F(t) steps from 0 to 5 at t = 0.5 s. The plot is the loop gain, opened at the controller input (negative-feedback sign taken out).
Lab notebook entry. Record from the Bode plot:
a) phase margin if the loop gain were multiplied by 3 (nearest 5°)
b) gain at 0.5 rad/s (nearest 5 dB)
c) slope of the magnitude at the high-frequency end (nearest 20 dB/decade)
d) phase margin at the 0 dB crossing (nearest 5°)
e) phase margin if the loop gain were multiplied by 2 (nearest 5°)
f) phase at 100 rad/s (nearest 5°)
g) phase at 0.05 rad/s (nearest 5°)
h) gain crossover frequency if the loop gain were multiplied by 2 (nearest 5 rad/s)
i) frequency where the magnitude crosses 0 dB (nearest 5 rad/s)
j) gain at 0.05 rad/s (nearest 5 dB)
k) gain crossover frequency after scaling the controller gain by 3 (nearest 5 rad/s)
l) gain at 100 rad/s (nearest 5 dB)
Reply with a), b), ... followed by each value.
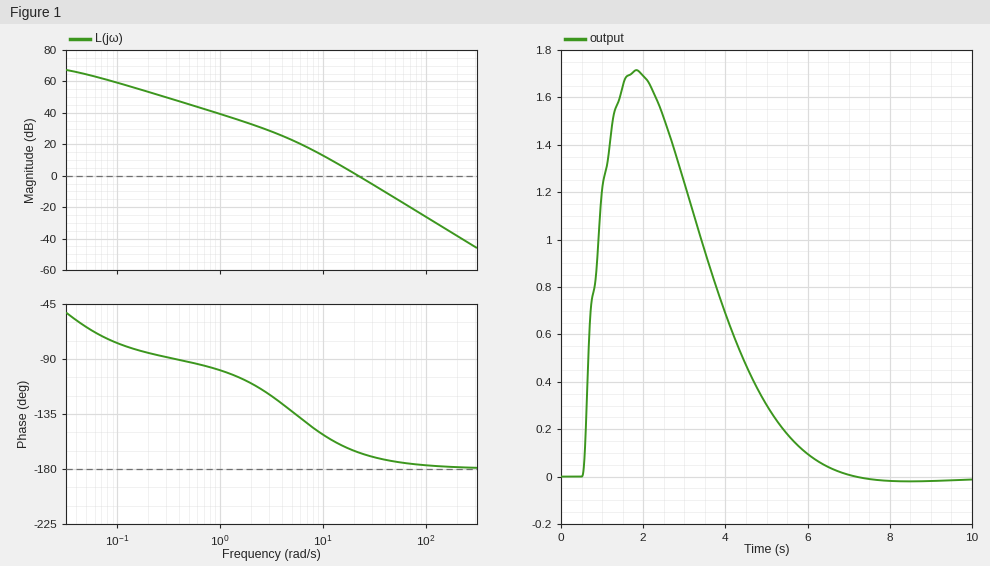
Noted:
a) 10°
b) 45 dB
c) -40 dB/decade
d) 15°
e) 10°
f) -175°
g) -65°
h) 30 rad/s
i) 20 rad/s
j) 65 dB
k) 40 rad/s
l) -25 dB
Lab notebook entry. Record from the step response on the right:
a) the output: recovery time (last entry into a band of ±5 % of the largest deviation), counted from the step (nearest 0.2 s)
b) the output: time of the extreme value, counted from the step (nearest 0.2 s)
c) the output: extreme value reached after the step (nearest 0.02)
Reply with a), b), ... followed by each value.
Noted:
a) 5.6 s
b) 1.4 s
c) 1.72
